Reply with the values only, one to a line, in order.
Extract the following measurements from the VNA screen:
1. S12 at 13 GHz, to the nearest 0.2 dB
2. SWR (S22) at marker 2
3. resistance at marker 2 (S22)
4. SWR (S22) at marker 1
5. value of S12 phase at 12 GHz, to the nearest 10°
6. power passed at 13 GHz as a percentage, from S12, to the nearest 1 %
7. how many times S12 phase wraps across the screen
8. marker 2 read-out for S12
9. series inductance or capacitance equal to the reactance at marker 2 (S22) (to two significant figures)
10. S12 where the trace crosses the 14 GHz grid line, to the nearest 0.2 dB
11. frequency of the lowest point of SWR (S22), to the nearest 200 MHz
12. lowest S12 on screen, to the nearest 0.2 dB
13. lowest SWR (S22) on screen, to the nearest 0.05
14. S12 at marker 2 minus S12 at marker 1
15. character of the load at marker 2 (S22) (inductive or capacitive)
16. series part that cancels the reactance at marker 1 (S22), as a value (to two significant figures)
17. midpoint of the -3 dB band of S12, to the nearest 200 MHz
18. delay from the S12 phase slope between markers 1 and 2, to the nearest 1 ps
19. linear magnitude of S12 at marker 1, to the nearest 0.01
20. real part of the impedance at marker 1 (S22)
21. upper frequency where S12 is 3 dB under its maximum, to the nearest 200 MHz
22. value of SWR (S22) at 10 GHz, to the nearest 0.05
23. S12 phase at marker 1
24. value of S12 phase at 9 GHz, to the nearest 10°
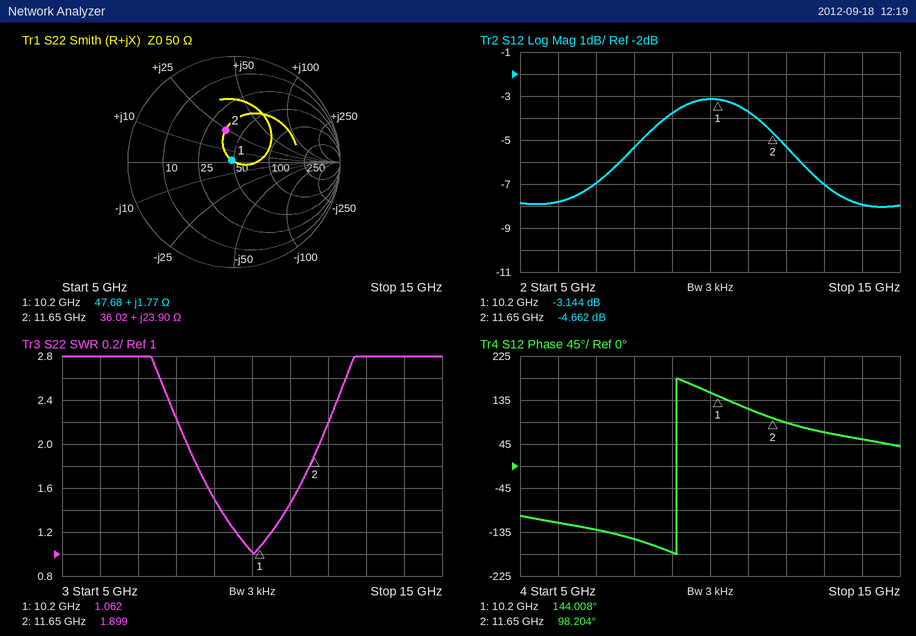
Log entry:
-7.0 dB
1.899
36.02 Ω
1.062
90°
20 %
1
-4.662 dB
330 pH
-8.0 dB
10.0 GHz
-8.0 dB
1.00
-1.518 dB
inductive
8.8 pF
10.0 GHz
88 ps
0.70
47.68 Ω
12.4 GHz
1.00
144.008°
-180°
